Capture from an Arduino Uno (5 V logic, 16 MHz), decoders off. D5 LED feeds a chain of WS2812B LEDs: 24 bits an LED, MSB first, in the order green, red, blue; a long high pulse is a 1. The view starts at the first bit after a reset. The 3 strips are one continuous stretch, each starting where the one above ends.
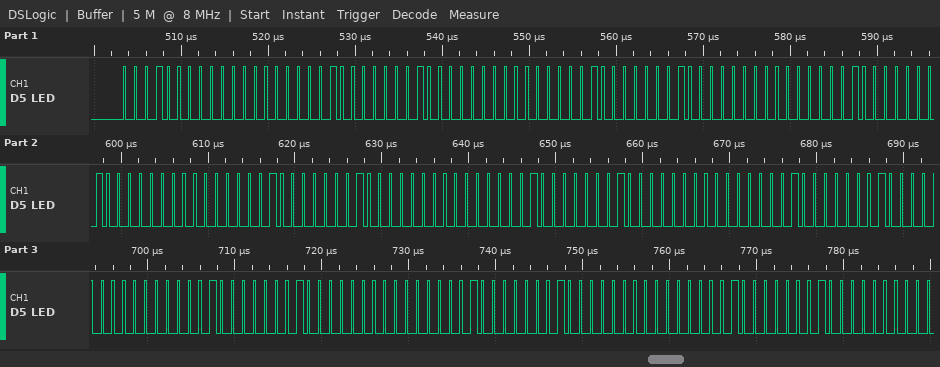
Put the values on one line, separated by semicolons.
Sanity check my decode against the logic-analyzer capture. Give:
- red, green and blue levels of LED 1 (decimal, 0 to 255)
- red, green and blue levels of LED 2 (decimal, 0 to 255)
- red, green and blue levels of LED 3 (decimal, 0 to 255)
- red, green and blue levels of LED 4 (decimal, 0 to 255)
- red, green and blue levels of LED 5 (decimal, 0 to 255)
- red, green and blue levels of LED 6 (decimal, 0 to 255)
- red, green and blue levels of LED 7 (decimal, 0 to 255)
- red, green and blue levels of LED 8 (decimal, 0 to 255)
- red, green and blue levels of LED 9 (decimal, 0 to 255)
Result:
0, 16, 16; 0, 16, 16; 0, 16, 16; 0, 16, 16; 0, 16, 16; 0, 16, 16; 0, 16, 16; 0, 16, 16; 0, 16, 16
